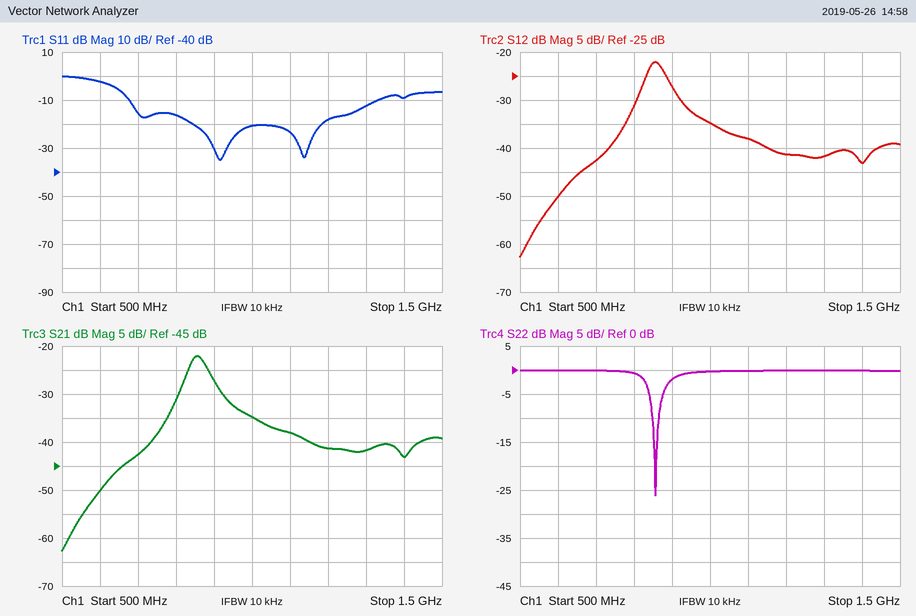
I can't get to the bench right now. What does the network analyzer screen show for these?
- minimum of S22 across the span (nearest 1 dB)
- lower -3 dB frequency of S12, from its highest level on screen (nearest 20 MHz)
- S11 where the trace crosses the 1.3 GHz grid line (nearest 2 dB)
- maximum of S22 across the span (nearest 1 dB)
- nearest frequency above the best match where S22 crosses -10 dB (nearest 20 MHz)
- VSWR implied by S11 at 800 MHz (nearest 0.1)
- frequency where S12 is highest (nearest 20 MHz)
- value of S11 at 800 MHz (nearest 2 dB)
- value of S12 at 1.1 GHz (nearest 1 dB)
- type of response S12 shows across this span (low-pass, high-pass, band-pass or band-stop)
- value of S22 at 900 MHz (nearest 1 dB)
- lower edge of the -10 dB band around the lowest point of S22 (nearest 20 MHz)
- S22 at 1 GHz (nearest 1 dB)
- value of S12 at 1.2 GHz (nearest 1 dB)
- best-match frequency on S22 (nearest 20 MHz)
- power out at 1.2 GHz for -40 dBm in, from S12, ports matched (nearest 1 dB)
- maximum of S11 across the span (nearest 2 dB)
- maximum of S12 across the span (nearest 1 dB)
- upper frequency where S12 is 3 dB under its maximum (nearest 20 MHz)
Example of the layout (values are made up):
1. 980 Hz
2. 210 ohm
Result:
1. -26 dB
2. 840 MHz
3. -12 dB
4. 0 dB
5. 860 MHz
6. 1.4
7. 860 MHz
8. -16 dB
9. -38 dB
10. band-pass
11. -2 dB
12. 840 MHz
13. 0 dB
14. -41 dB
15. 860 MHz
16. -81 dBm
17. 0 dB
18. -22 dB
19. 880 MHz
